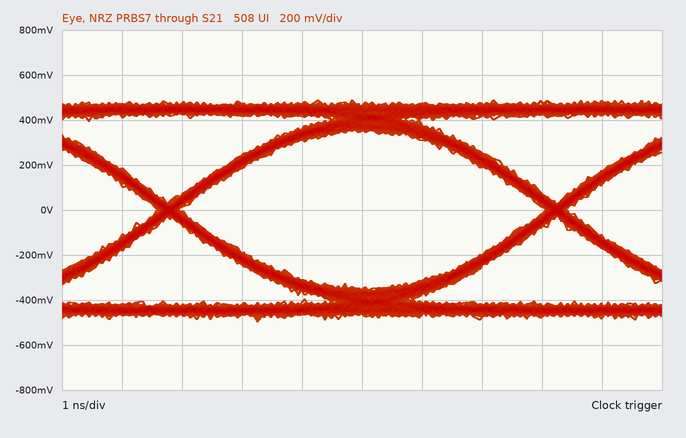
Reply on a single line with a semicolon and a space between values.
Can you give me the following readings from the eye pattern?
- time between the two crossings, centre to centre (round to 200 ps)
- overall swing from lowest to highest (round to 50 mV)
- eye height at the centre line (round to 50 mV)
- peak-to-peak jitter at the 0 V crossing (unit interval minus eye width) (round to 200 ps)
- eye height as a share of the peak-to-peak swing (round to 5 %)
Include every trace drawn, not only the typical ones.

6.4 ns; 1.00 V; 700 mV; 400 ps; 70 %
